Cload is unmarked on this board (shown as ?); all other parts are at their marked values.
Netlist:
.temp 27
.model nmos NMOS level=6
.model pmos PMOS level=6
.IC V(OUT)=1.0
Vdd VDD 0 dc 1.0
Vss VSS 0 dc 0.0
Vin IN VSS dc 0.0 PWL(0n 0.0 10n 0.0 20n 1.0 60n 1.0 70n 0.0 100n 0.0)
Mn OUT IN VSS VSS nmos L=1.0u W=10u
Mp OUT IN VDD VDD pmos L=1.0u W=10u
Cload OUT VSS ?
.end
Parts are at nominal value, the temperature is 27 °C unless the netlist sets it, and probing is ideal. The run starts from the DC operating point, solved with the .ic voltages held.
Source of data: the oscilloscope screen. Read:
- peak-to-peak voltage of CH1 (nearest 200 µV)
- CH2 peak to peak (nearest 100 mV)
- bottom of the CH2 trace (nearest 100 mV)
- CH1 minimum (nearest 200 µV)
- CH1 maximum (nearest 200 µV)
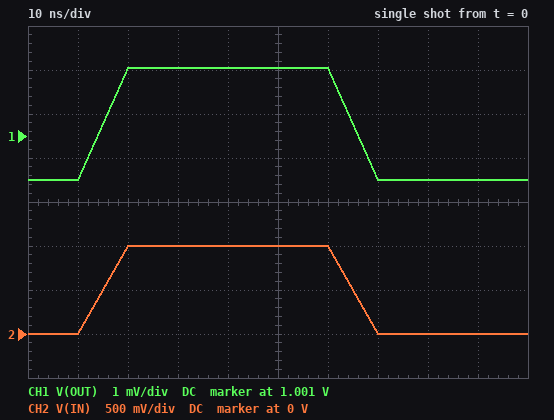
2.6 mV
1.0 V
0 V
1.0000 V
1.0026 V
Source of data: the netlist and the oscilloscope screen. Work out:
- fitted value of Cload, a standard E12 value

2.2 pF
